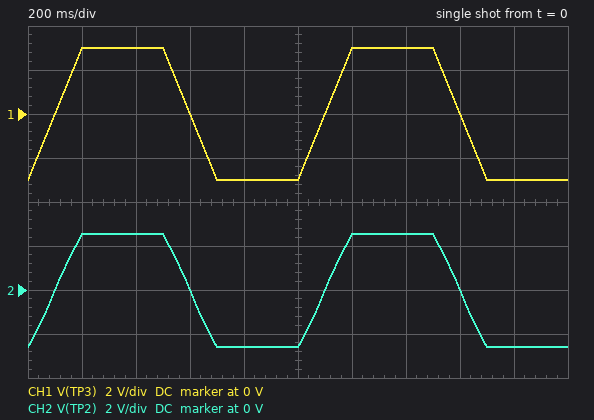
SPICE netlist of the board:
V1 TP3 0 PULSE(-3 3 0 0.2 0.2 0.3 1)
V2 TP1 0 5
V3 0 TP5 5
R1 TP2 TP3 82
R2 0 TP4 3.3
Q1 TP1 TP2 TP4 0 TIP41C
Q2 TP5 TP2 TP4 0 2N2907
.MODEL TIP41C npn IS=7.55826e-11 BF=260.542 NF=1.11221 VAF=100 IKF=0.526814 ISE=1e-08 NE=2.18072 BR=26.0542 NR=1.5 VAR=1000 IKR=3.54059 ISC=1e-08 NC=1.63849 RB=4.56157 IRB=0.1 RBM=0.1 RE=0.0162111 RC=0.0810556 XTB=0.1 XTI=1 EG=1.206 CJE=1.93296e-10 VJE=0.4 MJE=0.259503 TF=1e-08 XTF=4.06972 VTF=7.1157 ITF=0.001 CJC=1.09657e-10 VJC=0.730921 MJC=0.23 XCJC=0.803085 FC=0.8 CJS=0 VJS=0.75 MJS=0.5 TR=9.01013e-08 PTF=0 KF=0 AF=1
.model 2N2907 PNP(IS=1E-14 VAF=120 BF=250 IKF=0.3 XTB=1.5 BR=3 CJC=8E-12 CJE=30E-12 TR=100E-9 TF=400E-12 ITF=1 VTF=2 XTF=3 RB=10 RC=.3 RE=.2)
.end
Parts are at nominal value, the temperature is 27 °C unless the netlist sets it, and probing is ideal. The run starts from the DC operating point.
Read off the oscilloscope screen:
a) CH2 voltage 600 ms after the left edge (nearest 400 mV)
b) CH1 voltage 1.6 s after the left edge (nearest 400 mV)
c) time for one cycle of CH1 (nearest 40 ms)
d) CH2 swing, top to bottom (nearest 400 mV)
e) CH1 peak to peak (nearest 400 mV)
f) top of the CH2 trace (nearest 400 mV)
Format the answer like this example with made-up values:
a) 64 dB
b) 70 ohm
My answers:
a) 0 V
b) 0 V
c) 1.00 s
d) 5.2 V
e) 6.0 V
f) 2.4 V
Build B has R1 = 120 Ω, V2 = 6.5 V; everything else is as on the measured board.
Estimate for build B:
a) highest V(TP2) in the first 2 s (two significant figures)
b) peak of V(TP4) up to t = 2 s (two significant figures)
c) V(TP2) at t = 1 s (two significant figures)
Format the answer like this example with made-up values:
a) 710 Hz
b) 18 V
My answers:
a) 2.4 V
b) 1.7 V
c) -2.5 V
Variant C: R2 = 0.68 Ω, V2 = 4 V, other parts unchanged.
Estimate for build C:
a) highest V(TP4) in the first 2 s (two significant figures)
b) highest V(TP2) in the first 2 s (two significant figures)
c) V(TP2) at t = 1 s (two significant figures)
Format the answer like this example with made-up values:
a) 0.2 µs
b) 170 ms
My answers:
a) 820 mV
b) 1.6 V
c) -1.8 V
